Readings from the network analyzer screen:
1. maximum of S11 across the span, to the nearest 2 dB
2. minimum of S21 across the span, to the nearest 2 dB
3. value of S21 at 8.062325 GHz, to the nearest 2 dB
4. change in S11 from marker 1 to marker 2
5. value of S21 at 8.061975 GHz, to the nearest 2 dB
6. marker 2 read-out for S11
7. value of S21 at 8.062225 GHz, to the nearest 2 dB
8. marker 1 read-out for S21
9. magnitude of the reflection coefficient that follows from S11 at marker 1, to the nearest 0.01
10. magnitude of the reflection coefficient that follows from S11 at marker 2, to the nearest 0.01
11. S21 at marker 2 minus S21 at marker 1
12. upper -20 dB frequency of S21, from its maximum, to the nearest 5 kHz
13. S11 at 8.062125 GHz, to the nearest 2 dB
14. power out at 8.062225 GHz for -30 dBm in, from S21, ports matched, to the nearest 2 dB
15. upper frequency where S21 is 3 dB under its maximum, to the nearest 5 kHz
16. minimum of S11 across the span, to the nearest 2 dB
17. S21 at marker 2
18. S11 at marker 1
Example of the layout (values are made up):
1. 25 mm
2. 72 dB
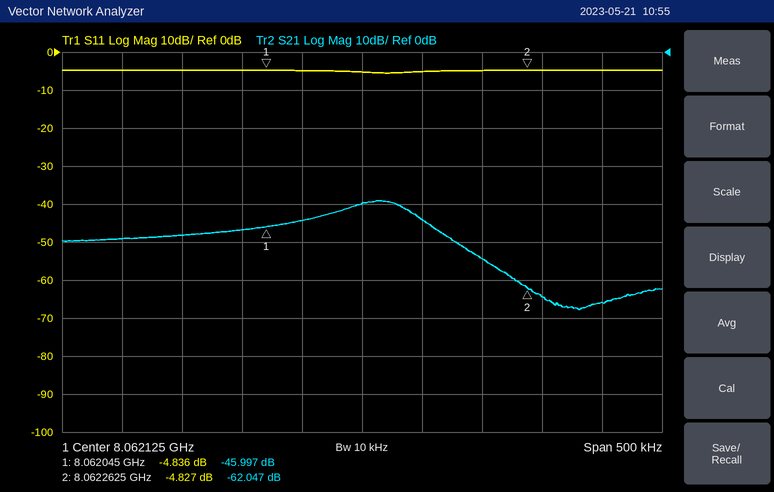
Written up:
1. -4 dB
2. -68 dB
3. -66 dB
4. 0.009 dB
5. -48 dB
6. -4.827 dB
7. -54 dB
8. -45.997 dB
9. 0.57
10. 0.57
11. -16.050 dB
12. 8.062250 GHz
13. -6 dB
14. -84 dBm
15. 8.062165 GHz
16. -6 dB
17. -62.047 dB
18. -4.836 dB
